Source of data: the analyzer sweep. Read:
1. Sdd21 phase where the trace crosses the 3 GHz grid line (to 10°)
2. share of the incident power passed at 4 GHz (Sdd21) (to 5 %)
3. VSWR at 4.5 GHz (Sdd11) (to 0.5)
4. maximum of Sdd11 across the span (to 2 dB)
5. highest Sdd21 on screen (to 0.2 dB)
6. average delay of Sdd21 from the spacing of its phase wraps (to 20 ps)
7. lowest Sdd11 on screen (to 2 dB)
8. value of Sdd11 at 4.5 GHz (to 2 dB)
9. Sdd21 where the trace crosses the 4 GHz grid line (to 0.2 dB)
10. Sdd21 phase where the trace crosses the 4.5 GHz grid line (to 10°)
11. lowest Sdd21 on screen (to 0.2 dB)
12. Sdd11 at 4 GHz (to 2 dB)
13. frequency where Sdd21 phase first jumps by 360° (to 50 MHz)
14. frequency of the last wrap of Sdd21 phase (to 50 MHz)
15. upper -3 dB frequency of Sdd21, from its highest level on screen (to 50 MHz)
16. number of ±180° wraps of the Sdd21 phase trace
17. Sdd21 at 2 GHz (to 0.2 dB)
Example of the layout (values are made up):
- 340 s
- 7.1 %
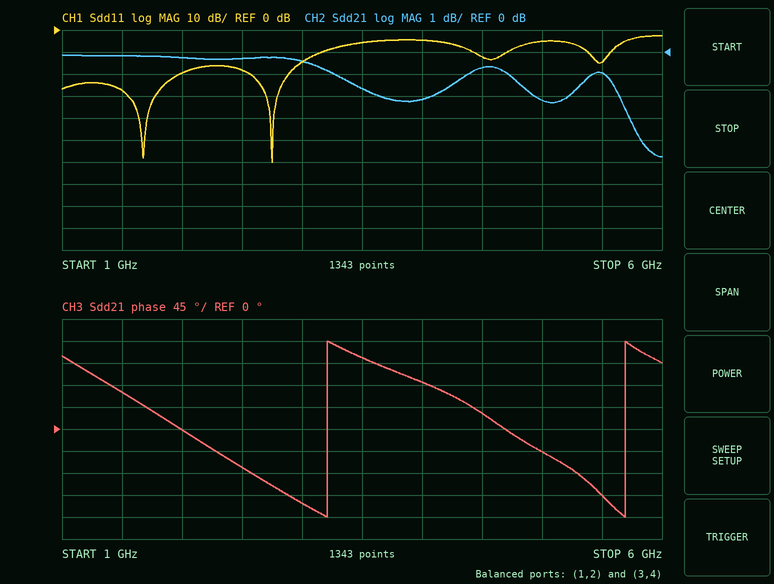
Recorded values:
- -150°
- 60 %
- 1.5
- -2 dB
- -0.2 dB
- 400 ps
- -60 dB
- -12 dB
- -2.2 dB
- 30°
- -4.8 dB
- -4 dB
- 3.20 GHz
- 5.70 GHz
- 5.75 GHz
- 2
- -0.2 dB
